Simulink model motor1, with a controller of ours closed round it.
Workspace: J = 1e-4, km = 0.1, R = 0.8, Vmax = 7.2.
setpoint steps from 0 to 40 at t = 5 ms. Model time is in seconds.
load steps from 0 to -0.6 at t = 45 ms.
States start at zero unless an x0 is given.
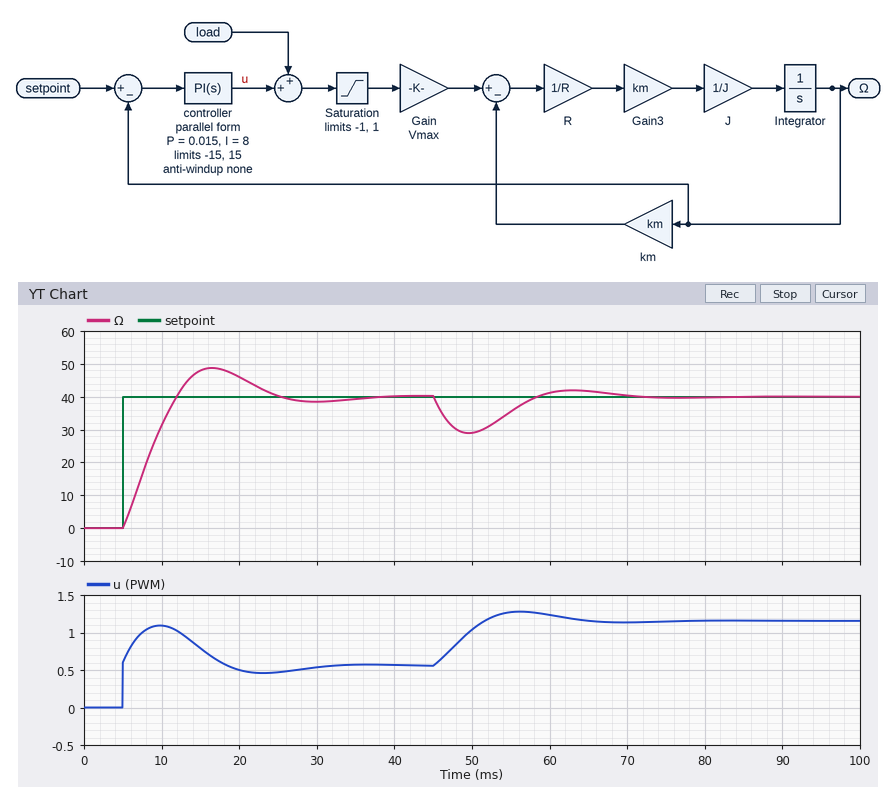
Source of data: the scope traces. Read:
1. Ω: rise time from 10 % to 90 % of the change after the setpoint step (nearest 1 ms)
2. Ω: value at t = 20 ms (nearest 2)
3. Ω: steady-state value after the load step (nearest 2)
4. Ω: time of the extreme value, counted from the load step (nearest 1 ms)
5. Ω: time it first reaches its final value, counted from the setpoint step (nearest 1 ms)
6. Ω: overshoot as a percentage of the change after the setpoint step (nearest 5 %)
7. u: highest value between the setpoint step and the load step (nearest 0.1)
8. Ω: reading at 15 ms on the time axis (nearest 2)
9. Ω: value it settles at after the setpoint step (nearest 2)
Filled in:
5 ms
46
40
5 ms
7 ms
20 %
1.1
48
40
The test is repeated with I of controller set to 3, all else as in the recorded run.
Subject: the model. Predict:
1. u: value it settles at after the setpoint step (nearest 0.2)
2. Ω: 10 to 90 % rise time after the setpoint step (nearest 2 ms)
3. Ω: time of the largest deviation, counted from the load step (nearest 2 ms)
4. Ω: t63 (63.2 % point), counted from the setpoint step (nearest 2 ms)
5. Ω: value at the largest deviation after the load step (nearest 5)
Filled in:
0.6
10 ms
6 ms
6 ms
25
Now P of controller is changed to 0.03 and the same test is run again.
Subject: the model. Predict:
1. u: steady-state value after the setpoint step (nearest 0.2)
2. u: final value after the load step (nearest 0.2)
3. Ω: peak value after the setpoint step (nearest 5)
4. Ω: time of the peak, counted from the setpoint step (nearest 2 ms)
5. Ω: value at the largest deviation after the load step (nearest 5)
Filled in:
0.6
1.2
45
10 ms
30
